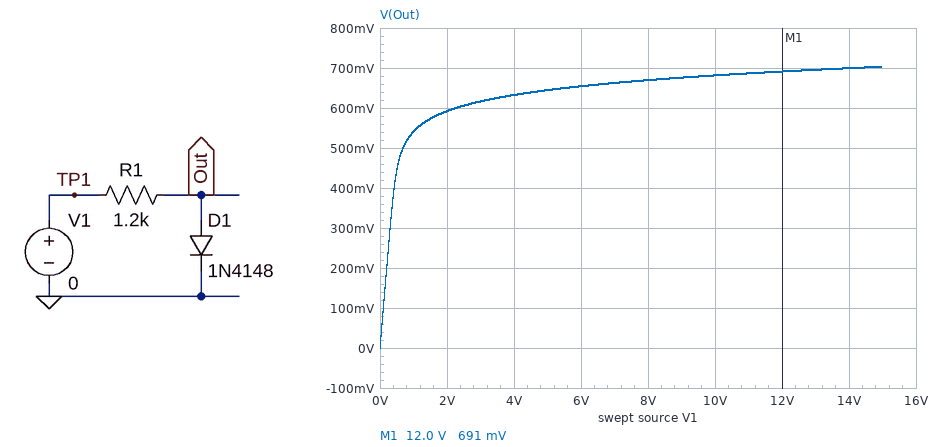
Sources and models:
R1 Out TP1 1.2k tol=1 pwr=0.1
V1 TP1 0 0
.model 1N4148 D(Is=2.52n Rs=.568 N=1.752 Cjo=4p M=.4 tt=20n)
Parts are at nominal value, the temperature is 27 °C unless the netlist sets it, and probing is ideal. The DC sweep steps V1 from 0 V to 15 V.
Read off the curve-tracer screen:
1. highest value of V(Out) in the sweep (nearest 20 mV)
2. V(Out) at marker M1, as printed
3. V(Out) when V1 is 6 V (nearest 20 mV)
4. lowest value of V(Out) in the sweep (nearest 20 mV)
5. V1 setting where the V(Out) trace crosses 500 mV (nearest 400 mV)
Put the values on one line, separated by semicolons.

700 mV; 691 mV; 660 mV; 0 V; 800 mV
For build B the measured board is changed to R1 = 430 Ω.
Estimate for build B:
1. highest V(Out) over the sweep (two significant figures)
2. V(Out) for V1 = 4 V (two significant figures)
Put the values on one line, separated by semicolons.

760 mV; 680 mV
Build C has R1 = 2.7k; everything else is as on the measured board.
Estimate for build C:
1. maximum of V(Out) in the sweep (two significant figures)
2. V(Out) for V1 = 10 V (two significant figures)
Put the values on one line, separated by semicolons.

660 mV; 640 mV
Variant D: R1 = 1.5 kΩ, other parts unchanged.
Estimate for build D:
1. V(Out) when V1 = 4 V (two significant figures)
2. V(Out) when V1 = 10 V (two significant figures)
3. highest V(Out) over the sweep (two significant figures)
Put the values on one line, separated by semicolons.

620 mV; 670 mV; 690 mV
